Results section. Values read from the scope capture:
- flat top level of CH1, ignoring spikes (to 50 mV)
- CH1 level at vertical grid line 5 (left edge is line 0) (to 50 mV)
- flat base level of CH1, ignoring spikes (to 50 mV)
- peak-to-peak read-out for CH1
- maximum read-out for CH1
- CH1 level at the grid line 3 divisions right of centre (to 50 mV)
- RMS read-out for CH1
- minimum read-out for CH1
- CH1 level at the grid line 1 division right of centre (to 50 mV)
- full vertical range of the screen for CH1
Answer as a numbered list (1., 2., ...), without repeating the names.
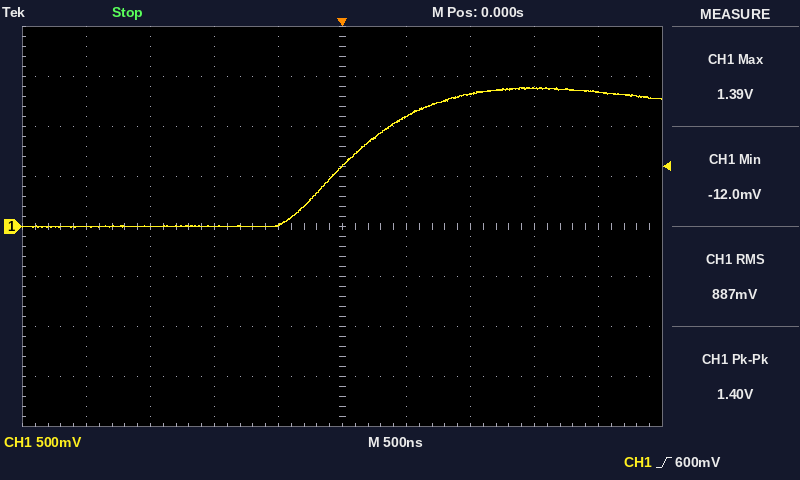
1. 1.35 V
2. 600 mV
3. 0 mV
4. 1.40 V
5. 1.39 V
6. 1.40 V
7. 887 mV
8. -12.0 mV
9. 1.10 V
10. 4 V
